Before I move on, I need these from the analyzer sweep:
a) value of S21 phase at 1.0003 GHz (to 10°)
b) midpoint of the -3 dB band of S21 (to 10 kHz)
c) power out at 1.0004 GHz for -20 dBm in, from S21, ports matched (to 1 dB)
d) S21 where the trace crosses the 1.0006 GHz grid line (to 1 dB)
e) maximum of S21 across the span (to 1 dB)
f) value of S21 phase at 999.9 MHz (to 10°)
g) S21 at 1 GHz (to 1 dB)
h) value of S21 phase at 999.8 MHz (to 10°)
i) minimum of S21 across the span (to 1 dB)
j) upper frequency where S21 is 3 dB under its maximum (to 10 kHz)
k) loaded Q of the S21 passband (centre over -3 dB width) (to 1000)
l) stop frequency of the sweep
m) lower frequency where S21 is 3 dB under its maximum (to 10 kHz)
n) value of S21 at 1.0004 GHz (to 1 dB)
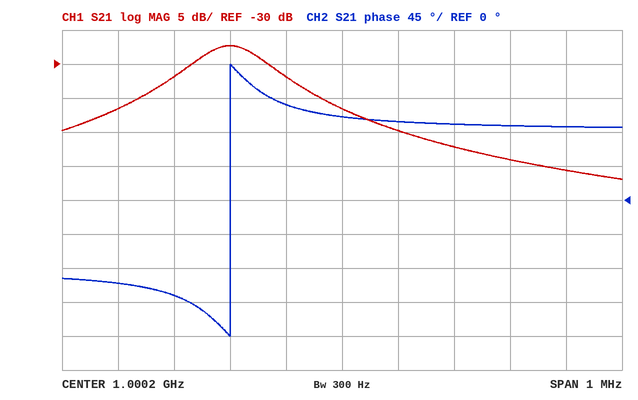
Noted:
100°
1.00000 GHz
-62 dBm
-46 dB
-27 dB
-130°
-27 dB
-110°
-47 dB
1.00007 GHz
7000
1.0007 GHz
999.93 MHz
-42 dB
